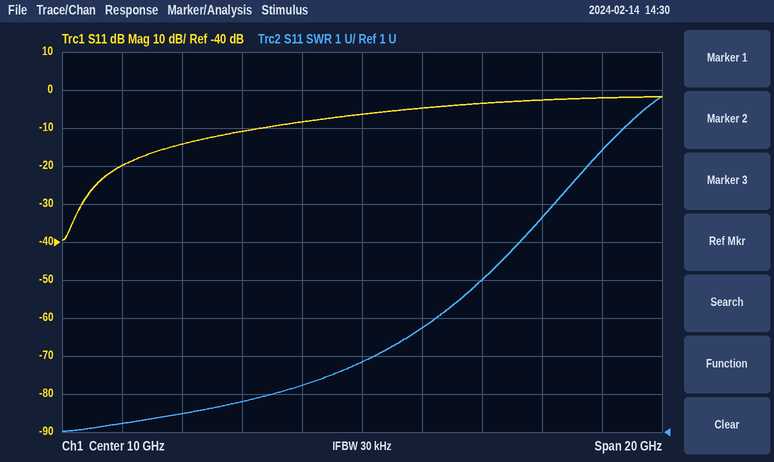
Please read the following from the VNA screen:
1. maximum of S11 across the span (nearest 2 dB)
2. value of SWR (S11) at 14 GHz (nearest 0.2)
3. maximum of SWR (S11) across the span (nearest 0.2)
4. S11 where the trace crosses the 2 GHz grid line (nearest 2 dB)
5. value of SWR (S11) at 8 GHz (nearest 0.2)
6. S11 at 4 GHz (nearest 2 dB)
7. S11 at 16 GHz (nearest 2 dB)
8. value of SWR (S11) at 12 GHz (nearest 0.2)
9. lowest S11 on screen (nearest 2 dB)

-2 dB
5.0
9.8
-20 dB
2.2
-14 dB
-2 dB
3.8
-40 dB
